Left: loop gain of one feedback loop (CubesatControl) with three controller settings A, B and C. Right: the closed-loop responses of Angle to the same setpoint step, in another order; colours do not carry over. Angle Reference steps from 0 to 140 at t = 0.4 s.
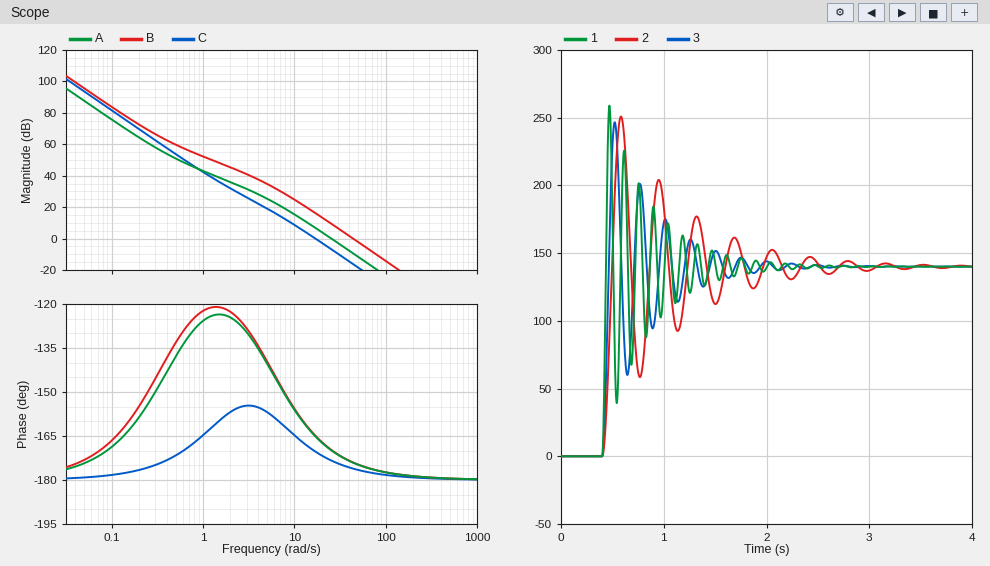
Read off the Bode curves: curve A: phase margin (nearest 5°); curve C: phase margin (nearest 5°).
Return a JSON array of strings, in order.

["10°", "10°"]
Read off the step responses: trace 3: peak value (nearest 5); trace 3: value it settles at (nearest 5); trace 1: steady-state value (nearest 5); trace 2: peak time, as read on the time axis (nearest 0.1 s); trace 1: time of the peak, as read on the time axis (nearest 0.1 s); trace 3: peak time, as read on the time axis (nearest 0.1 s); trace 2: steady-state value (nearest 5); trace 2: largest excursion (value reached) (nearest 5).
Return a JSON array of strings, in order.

["245", "140", "140", "0.6 s", "0.5 s", "0.5 s", "140", "250"]
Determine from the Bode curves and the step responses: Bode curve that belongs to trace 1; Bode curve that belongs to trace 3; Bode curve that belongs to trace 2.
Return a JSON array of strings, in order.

["B", "A", "C"]
